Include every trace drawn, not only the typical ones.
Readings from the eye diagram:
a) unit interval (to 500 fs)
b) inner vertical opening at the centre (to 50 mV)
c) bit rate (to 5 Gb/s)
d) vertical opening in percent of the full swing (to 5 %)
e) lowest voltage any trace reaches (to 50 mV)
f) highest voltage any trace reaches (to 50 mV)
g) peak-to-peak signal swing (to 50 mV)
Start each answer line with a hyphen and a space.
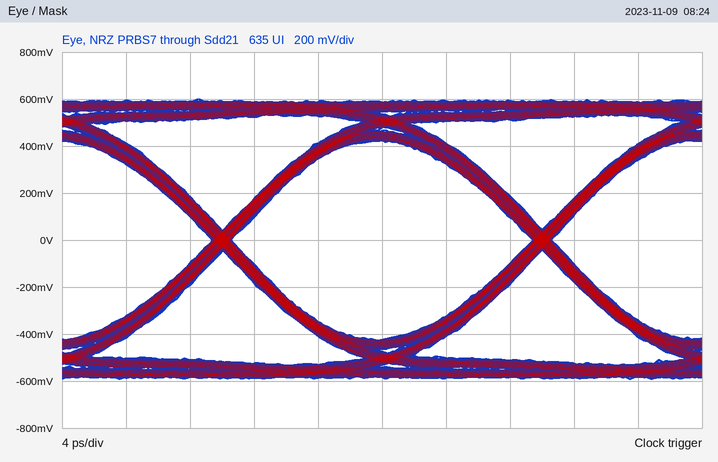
- 20.0 ps
- 850 mV
- 50 Gb/s
- 70 %
- -600 mV
- 600 mV
- 1.20 V
